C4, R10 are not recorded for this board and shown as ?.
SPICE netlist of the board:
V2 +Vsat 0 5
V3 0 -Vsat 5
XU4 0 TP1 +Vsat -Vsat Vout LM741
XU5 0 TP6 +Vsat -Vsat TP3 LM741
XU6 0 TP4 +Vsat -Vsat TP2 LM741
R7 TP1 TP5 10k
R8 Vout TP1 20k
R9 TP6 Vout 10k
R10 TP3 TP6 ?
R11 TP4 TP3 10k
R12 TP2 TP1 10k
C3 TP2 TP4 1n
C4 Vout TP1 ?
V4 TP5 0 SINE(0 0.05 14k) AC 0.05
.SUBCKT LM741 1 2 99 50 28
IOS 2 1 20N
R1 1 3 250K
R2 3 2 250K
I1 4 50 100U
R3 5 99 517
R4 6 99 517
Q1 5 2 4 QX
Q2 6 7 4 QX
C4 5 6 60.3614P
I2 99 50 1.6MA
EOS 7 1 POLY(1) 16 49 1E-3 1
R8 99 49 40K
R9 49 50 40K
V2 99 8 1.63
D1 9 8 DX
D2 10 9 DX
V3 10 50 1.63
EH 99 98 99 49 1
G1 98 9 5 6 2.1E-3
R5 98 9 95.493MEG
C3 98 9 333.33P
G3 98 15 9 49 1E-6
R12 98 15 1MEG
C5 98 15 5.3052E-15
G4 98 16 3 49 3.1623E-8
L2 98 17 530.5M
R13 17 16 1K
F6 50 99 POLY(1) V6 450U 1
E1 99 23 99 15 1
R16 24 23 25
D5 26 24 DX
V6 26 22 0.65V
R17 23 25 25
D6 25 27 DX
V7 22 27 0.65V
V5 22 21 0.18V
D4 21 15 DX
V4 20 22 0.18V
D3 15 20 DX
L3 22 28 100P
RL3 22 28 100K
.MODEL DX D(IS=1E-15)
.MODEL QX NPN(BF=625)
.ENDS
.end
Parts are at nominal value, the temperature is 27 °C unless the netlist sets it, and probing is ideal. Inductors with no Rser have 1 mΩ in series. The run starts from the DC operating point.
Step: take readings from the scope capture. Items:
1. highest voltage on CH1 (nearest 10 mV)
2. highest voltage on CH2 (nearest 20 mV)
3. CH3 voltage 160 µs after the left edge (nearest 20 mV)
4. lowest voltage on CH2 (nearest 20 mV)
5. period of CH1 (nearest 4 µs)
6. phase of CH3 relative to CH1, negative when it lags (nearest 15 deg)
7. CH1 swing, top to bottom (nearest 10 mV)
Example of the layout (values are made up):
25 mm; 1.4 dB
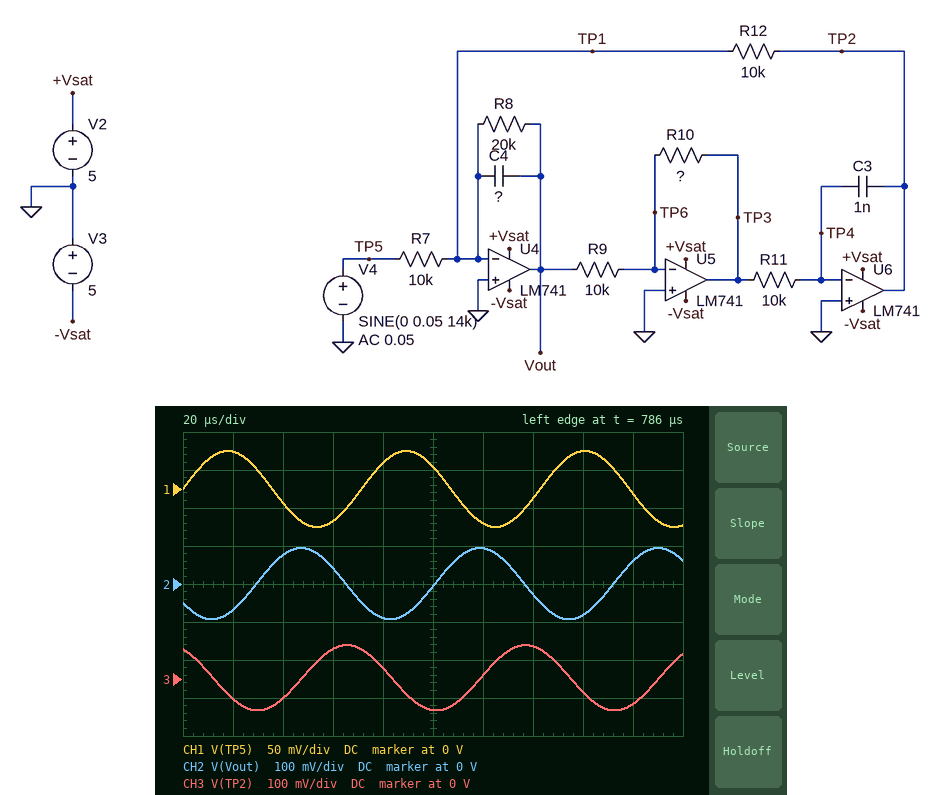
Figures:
50 mV; 100 mV; -40 mV; -100 mV; 72 µs; 120 deg; 100 mV
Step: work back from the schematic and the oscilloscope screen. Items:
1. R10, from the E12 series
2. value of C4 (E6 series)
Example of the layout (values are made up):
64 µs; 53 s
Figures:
8.2 kΩ; 680 pF
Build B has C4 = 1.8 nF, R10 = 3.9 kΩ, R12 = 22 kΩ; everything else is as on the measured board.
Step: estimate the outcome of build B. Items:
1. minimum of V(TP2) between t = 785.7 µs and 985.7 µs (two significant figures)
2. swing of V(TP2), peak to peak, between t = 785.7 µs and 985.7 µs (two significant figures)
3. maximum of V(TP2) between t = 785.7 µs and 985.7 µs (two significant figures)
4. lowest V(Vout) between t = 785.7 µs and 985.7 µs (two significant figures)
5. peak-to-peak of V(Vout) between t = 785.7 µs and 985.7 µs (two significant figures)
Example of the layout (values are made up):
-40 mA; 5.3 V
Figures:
-7.5 mV; 29 mV; 22 mV; -34 mV; 67 mV
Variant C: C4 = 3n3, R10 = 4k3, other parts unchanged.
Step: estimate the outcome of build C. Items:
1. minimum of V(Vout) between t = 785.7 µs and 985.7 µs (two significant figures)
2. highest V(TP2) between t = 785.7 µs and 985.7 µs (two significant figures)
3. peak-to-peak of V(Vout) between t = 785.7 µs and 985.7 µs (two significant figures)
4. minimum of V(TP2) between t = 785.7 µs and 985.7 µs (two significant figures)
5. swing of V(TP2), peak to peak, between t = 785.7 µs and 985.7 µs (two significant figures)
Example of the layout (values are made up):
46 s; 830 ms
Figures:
-20 mV; 13 mV; 40 mV; -6.0 mV; 19 mV
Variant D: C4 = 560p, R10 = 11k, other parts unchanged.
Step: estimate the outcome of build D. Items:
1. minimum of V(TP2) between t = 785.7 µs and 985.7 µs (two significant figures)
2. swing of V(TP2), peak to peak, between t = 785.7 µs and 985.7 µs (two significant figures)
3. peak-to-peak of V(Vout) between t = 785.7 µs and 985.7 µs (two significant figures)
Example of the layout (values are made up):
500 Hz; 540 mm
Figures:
-72 mV; 150 mV; 120 mV
